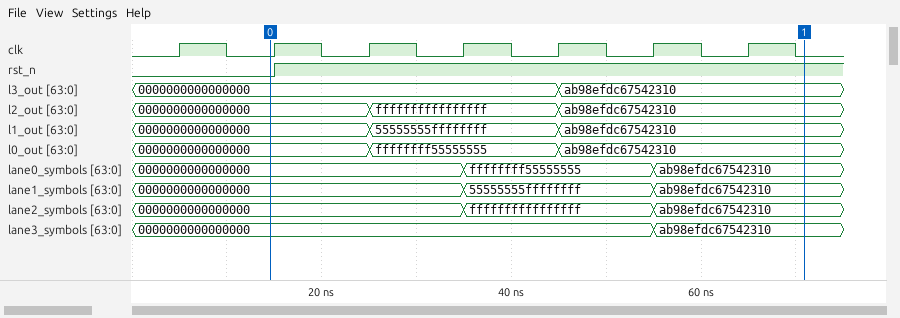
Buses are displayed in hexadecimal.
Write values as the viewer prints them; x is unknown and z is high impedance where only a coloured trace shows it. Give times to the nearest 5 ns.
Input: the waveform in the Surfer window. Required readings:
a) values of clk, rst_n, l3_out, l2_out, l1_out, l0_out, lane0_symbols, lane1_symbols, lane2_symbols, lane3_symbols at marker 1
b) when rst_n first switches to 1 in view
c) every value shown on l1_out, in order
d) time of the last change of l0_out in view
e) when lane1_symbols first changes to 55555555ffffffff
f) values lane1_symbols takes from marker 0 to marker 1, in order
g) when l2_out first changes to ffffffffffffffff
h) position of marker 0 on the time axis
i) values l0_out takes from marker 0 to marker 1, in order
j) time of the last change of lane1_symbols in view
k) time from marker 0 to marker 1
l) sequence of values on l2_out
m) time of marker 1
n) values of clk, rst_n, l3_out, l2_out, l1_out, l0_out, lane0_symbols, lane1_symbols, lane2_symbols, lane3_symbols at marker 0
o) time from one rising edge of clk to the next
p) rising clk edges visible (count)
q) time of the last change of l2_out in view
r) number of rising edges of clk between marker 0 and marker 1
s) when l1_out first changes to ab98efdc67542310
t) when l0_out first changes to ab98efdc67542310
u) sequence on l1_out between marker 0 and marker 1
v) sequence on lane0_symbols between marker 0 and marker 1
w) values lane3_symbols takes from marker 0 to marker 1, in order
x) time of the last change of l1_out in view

clk=0, rst_n=1, l3_out=ab98efdc67542310, l2_out=ab98efdc67542310, l1_out=ab98efdc67542310, l0_out=ab98efdc67542310, lane0_symbols=ab98efdc67542310, lane1_symbols=ab98efdc67542310, lane2_symbols=ab98efdc67542310, lane3_symbols=ab98efdc67542310
15 ns
0000000000000000, 55555555ffffffff, ab98efdc67542310
45 ns
35 ns
0000000000000000, 55555555ffffffff, ab98efdc67542310
25 ns
15 ns
0000000000000000, ffffffff55555555, ab98efdc67542310
55 ns
55 ns
0000000000000000, ffffffffffffffff, ab98efdc67542310
70 ns
clk=0, rst_n=0, l3_out=0000000000000000, l2_out=0000000000000000, l1_out=0000000000000000, l0_out=0000000000000000, lane0_symbols=0000000000000000, lane1_symbols=0000000000000000, lane2_symbols=0000000000000000, lane3_symbols=0000000000000000
10 ns
7
45 ns
6
45 ns
45 ns
0000000000000000, 55555555ffffffff, ab98efdc67542310
0000000000000000, ffffffff55555555, ab98efdc67542310
0000000000000000, ab98efdc67542310
45 ns
